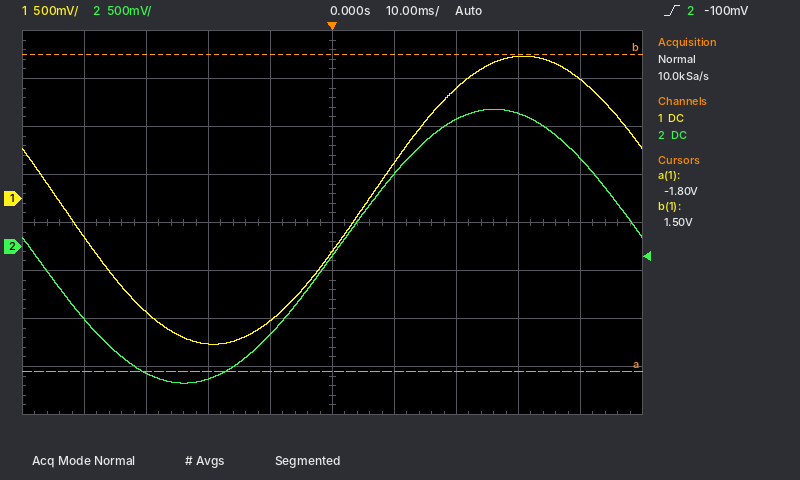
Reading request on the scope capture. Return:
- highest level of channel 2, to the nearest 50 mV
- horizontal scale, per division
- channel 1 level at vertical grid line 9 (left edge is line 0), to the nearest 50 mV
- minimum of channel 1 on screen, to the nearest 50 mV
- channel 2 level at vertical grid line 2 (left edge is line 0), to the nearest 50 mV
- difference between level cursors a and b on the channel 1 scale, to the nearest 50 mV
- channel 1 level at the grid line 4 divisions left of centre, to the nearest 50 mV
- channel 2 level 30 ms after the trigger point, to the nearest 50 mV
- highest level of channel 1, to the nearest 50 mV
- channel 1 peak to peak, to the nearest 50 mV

1.45 V
10 ms
1.25 V
-1.50 V
-1.30 V
3.30 V
-400 mV
1.40 V
1.50 V
3.00 V
